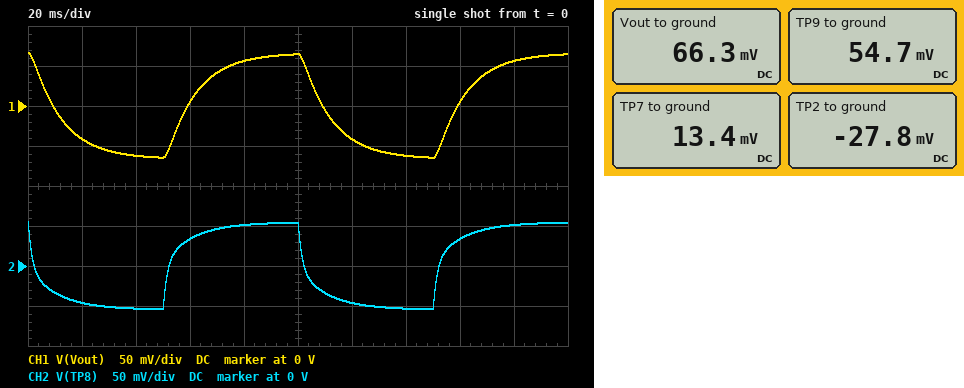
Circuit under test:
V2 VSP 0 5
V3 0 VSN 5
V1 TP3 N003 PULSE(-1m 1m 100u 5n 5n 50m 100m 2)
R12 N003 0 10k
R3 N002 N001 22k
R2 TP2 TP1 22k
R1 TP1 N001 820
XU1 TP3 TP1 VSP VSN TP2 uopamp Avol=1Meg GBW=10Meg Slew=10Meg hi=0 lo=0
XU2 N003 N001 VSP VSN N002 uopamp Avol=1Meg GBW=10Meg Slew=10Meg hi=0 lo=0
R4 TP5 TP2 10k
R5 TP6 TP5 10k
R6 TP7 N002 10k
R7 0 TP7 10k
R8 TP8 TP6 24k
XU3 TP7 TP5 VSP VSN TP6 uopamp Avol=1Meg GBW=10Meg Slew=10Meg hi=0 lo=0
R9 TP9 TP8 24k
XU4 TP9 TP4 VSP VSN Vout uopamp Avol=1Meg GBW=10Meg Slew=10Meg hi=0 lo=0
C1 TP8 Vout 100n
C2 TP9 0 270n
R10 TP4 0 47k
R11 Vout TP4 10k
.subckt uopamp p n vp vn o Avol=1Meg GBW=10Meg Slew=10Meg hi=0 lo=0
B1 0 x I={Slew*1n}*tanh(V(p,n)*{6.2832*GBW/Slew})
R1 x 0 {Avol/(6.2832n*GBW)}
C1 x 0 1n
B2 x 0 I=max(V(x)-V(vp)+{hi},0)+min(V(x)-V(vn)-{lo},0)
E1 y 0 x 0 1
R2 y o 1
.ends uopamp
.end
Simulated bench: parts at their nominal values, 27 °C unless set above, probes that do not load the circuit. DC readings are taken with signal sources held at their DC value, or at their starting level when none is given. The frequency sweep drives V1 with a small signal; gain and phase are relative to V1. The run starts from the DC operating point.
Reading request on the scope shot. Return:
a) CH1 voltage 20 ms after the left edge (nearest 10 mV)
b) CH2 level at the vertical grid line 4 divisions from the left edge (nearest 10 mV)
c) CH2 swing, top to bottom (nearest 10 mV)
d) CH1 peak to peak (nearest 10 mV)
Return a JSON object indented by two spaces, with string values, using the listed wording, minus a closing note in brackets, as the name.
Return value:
{
  "CH1 voltage 20 ms after the left edge": "-40 mV",
  "CH2 level at the vertical grid line 4 divisions from the left edge": "50 mV",
  "CH2 swing, top to bottom": "110 mV",
  "CH1 peak to peak": "130 mV"
}
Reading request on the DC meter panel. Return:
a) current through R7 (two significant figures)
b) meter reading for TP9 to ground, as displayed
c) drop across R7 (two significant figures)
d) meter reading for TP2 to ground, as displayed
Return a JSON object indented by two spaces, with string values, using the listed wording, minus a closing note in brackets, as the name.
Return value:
{
  "current through R7": "1.3 µA",
  "meter reading for TP9 to ground, as displayed": "54.7 mV",
  "drop across R7": "13 mV",
  "meter reading for TP2 to ground, as displayed": "-27.8 mV"
}
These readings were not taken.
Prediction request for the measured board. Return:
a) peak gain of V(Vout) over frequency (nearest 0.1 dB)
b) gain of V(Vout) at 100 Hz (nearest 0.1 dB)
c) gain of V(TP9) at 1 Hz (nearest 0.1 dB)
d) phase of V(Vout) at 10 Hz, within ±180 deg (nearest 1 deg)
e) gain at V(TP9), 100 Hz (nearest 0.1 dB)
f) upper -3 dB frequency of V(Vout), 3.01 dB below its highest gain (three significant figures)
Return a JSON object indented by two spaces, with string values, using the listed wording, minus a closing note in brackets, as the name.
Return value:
{
  "peak gain of V(Vout) over frequency": "36.4 dB",
  "gain of V(Vout) at 100 Hz": "17.0 dB",
  "gain of V(TP9) at 1 Hz": "34.7 dB",
  "phase of V(Vout) at 10 Hz, within ±180 deg": "140 deg",
  "gain at V(TP9), 100 Hz": "15.3 dB",
  "upper -3 dB frequency of V(Vout), 3.01 dB below its highest gain": "14.2 Hz"
}
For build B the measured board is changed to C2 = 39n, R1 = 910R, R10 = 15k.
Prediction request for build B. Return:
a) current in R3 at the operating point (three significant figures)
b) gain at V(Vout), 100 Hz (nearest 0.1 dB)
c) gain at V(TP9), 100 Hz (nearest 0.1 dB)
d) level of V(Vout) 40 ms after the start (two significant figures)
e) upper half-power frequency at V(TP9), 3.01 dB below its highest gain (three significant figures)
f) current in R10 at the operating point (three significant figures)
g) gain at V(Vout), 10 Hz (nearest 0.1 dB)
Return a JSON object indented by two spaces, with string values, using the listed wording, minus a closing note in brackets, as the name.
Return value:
{
  "current in R3 at the operating point": "1.10 µA",
  "gain at V(Vout), 100 Hz": "52.1 dB",
  "gain at V(TP9), 100 Hz": "47.6 dB",
  "level of V(Vout) 40 ms after the start": "-78 mV",
  "upper half-power frequency at V(TP9), 3.01 dB below its highest gain": "115 Hz",
  "current in R10 at the operating point": "3.29 µA",
  "gain at V(Vout), 10 Hz": "38.4 dB"
}
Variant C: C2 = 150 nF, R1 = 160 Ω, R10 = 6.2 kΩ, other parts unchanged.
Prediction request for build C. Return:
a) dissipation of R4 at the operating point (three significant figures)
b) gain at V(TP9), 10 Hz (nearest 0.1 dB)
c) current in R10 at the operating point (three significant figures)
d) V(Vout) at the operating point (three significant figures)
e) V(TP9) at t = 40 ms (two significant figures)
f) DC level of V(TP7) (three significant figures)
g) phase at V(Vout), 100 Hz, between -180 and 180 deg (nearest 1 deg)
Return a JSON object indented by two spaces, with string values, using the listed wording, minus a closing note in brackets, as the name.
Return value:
{
  "dissipation of R4 at the operating point": "4.29 µW",
  "gain at V(TP9), 10 Hz": "48.9 dB",
  "current in R10 at the operating point": "44.5 µA",
  "V(Vout) at the operating point": "721 mV",
  "V(TP9) at t = 40 ms": "-280 mV",
  "DC level of V(TP7)": "68.7 mV",
  "phase at V(Vout), 100 Hz, between -180 and 180 deg": "41 deg"
}
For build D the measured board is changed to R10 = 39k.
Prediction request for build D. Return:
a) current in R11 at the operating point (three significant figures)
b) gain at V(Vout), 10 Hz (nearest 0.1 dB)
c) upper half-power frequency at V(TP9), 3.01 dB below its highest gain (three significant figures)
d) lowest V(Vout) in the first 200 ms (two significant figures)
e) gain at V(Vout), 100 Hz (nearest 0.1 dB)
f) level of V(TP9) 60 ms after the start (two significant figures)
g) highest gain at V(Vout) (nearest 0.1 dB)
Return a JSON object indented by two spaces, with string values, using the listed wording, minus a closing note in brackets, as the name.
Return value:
{
  "current in R11 at the operating point": "1.40 µA",
  "gain at V(Vout), 10 Hz": "35.0 dB",
  "upper half-power frequency at V(TP9), 3.01 dB below its highest gain": "14.3 Hz",
  "lowest V(Vout) in the first 200 ms": "-67 mV",
  "gain at V(Vout), 100 Hz": "17.4 dB",
  "level of V(TP9) 60 ms after the start": "4.4 mV",
  "highest gain at V(Vout)": "36.7 dB"
}
